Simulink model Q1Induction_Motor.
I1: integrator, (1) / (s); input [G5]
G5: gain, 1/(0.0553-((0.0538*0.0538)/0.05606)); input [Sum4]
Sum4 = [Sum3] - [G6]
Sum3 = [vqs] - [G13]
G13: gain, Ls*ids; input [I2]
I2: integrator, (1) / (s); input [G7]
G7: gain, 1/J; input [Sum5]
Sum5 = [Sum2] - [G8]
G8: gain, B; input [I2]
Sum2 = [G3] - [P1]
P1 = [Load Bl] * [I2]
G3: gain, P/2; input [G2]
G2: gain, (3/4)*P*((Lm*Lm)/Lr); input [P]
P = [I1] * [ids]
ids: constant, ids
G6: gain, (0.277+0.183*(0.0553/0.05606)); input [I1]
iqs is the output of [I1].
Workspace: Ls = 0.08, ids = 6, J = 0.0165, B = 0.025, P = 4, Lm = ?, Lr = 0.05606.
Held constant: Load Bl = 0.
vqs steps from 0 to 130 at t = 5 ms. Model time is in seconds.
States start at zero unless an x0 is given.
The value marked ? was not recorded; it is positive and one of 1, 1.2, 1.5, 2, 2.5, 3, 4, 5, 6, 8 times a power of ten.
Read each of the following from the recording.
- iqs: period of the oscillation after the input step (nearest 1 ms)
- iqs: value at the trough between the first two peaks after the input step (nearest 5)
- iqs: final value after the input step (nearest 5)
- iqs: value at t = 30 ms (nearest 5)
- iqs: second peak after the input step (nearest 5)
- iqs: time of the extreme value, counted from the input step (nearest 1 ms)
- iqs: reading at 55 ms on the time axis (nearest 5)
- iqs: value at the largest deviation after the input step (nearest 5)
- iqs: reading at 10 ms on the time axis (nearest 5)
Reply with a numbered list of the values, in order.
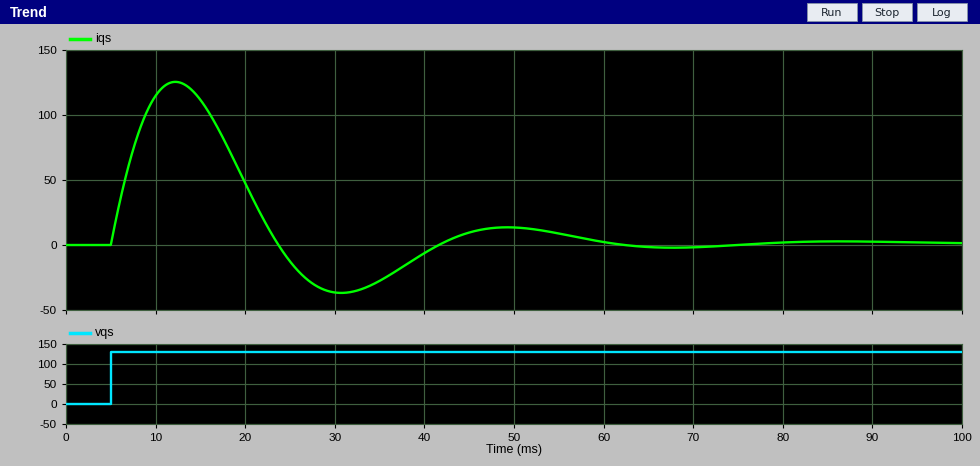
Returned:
1. 37 ms
2. -35
3. 0
4. -35
5. 15
6. 7 ms
7. 10
8. 125
9. 115
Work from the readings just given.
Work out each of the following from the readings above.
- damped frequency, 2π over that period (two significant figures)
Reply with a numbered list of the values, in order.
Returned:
1. 0.17 rad/ms
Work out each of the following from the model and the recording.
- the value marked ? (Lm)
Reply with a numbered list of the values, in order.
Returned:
1. 0.08
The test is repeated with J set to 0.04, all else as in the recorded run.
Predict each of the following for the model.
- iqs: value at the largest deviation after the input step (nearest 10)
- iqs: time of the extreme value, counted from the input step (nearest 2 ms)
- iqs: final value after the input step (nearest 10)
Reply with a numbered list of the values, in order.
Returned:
1. 160
2. 10 ms
3. 0
